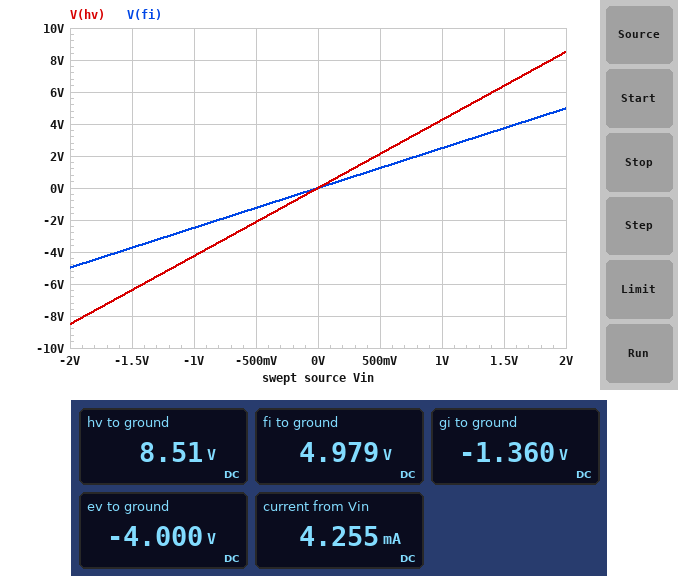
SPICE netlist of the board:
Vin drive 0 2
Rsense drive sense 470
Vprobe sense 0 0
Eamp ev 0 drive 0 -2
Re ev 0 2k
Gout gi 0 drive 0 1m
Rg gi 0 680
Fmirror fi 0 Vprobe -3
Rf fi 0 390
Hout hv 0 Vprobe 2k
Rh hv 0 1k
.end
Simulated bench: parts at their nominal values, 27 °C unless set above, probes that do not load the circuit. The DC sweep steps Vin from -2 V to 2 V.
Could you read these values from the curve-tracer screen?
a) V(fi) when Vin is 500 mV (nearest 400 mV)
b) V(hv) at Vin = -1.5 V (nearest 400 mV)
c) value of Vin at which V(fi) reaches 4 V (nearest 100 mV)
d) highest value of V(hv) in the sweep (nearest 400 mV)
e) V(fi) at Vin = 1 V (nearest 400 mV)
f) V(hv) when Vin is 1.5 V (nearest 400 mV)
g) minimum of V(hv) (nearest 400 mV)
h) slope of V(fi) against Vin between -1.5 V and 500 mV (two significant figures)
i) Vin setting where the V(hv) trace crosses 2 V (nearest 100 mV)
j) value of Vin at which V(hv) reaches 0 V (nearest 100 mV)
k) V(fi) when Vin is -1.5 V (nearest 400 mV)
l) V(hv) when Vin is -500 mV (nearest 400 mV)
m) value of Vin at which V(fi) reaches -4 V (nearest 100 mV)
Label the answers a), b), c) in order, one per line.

a) 1.2 V
b) -6.4 V
c) 1.6 V
d) 8.4 V
e) 2.4 V
f) 6.4 V
g) -8.4 V
h) 2.5 V/V
i) 500 mV
j) 0 V
k) -3.6 V
l) -2.0 V
m) -1.6 V
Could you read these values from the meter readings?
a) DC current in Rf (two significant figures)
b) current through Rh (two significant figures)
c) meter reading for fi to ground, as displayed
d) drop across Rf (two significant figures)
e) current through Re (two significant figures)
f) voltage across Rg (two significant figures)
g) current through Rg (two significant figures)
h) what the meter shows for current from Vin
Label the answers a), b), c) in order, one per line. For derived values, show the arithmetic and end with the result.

a) (4.979 V) / 390 Ω = 13 mA
b) (8.51 V) / 1 kΩ = 8.5 mA
c) 4.979 V
d) 4.979 V = 5.0 V
e) (0 V - (-4 V)) / 2 kΩ = 2.0 mA
f) 0 V - (-1.36 V) = 1.4 V
g) (0 V - (-1.36 V)) / 680 Ω = 2.0 mA
h) 4.255 mA
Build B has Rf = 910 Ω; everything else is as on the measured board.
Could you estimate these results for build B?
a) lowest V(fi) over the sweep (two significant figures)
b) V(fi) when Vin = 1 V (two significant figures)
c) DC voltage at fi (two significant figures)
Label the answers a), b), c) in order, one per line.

a) -12 V
b) 5.8 V
c) 12 V
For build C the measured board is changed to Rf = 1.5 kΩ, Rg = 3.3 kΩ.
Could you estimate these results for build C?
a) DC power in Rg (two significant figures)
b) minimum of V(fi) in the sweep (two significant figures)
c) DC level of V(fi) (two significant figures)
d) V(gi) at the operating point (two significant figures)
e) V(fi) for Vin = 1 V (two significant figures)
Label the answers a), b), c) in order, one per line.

a) 13 mW
b) -19 V
c) 19 V
d) -6.6 V
e) 9.6 V
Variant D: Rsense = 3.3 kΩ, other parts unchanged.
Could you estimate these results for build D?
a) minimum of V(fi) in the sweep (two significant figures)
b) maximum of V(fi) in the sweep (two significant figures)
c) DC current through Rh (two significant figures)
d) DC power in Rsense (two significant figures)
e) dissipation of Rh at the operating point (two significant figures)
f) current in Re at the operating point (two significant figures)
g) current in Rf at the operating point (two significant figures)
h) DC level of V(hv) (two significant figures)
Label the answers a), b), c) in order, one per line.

a) -710 mV
b) 710 mV
c) 1.2 mA
d) 1.2 mW
e) 1.5 mW
f) 2.0 mA
g) 1.8 mA
h) 1.2 V
